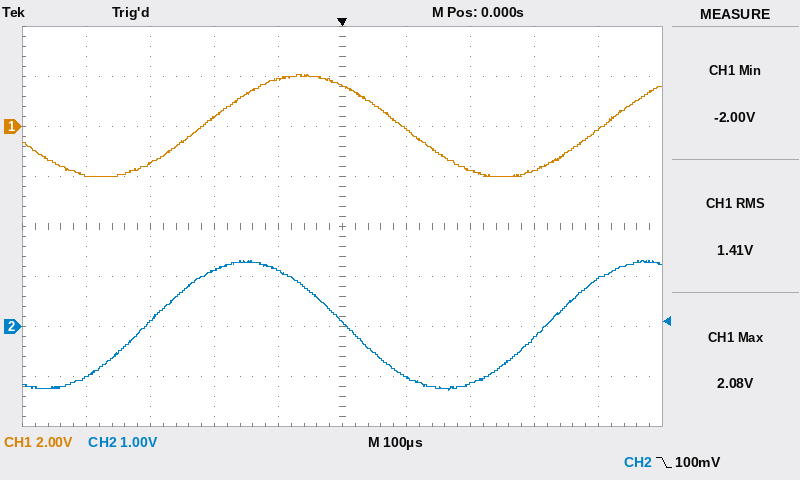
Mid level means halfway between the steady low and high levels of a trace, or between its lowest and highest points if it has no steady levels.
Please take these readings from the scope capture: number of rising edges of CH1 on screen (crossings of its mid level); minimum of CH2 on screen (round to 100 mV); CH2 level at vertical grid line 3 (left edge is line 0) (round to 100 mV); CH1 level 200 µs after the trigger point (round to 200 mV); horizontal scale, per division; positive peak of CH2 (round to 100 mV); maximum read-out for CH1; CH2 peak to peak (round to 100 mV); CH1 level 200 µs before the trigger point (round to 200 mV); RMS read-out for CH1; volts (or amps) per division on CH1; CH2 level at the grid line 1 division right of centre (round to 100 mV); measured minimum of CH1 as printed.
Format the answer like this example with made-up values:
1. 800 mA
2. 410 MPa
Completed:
1. 2
2. -1.3 V
3. 1.1 V
4. -1.8 V
5. 100 µs
6. 1.3 V
7. 2.08 V
8. 2.6 V
9. 400 mV
10. 1.41 V
11. 2 V
12. -1.0 V
13. -2.00 V
